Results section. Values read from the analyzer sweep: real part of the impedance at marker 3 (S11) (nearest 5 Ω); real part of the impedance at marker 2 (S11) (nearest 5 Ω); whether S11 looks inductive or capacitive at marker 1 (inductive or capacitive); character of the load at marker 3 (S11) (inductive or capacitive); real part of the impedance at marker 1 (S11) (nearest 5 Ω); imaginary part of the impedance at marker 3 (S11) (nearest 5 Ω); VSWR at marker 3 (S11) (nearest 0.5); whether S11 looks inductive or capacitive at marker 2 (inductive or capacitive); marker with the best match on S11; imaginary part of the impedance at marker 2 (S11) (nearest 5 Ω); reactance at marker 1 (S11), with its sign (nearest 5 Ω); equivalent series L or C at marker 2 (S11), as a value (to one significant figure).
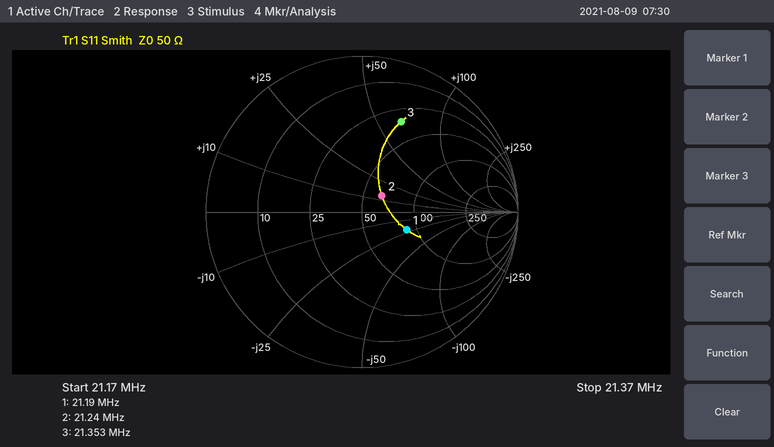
35 Ω
65 Ω
capacitive
inductive
85 Ω
+65 Ω
4.5
inductive
marker 2
+15 Ω
-20 Ω
100 nH
